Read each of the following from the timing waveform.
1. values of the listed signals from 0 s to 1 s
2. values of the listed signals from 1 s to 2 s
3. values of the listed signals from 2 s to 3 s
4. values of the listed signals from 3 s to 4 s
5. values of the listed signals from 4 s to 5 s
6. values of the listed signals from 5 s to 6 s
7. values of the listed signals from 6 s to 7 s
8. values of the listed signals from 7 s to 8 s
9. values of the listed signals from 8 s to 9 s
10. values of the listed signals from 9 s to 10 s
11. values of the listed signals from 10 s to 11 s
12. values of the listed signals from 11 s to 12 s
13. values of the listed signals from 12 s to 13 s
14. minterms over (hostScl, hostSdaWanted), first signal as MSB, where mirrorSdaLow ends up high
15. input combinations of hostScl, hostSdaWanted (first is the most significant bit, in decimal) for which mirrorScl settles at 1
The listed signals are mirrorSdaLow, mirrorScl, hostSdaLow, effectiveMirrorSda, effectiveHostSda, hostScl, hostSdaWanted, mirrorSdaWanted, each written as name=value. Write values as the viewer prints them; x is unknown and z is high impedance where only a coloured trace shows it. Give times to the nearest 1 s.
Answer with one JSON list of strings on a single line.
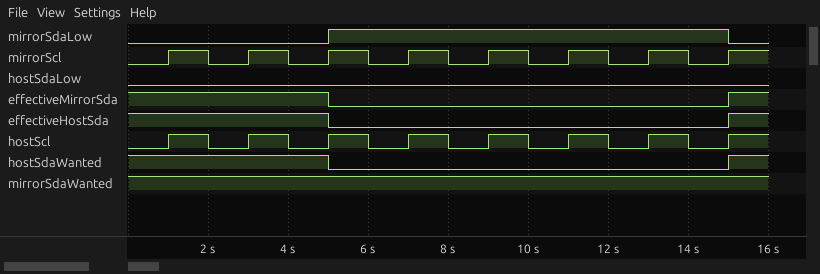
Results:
["mirrorSdaLow=0, mirrorScl=0, hostSdaLow=0, effectiveMirrorSda=1, effectiveHostSda=1, hostScl=0, hostSdaWanted=1, mirrorSdaWanted=1", "mirrorSdaLow=0, mirrorScl=1, hostSdaLow=0, effectiveMirrorSda=1, effectiveHostSda=1, hostScl=1, hostSdaWanted=1, mirrorSdaWanted=1", "mirrorSdaLow=0, mirrorScl=0, hostSdaLow=0, effectiveMirrorSda=1, effectiveHostSda=1, hostScl=0, hostSdaWanted=1, mirrorSdaWanted=1", "mirrorSdaLow=0, mirrorScl=1, hostSdaLow=0, effectiveMirrorSda=1, effectiveHostSda=1, hostScl=1, hostSdaWanted=1, mirrorSdaWanted=1", "mirrorSdaLow=0, mirrorScl=0, hostSdaLow=0, effectiveMirrorSda=1, effectiveHostSda=1, hostScl=0, hostSdaWanted=1, mirrorSdaWanted=1", "mirrorSdaLow=1, mirrorScl=1, hostSdaLow=0, effectiveMirrorSda=0, effectiveHostSda=0, hostScl=1, hostSdaWanted=0, mirrorSdaWanted=1", "mirrorSdaLow=1, mirrorScl=0, hostSdaLow=0, effectiveMirrorSda=0, effectiveHostSda=0, hostScl=0, hostSdaWanted=0, mirrorSdaWanted=1", "mirrorSdaLow=1, mirrorScl=1, hostSdaLow=0, effectiveMirrorSda=0, effectiveHostSda=0, hostScl=1, hostSdaWanted=0, mirrorSdaWanted=1", "mirrorSdaLow=1, mirrorScl=0, hostSdaLow=0, effectiveMirrorSda=0, effectiveHostSda=0, hostScl=0, hostSdaWanted=0, mirrorSdaWanted=1", "mirrorSdaLow=1, mirrorScl=1, hostSdaLow=0, effectiveMirrorSda=0, effectiveHostSda=0, hostScl=1, hostSdaWanted=0, mirrorSdaWanted=1", "mirrorSdaLow=1, mirrorScl=0, hostSdaLow=0, effectiveMirrorSda=0, effectiveHostSda=0, hostScl=0, hostSdaWanted=0, mirrorSdaWanted=1", "mirrorSdaLow=1, mirrorScl=1, hostSdaLow=0, effectiveMirrorSda=0, effectiveHostSda=0, hostScl=1, hostSdaWanted=0, mirrorSdaWanted=1", "mirrorSdaLow=1, mirrorScl=0, hostSdaLow=0, effectiveMirrorSda=0, effectiveHostSda=0, hostScl=0, hostSdaWanted=0, mirrorSdaWanted=1", "0, 2", "2, 3"]
